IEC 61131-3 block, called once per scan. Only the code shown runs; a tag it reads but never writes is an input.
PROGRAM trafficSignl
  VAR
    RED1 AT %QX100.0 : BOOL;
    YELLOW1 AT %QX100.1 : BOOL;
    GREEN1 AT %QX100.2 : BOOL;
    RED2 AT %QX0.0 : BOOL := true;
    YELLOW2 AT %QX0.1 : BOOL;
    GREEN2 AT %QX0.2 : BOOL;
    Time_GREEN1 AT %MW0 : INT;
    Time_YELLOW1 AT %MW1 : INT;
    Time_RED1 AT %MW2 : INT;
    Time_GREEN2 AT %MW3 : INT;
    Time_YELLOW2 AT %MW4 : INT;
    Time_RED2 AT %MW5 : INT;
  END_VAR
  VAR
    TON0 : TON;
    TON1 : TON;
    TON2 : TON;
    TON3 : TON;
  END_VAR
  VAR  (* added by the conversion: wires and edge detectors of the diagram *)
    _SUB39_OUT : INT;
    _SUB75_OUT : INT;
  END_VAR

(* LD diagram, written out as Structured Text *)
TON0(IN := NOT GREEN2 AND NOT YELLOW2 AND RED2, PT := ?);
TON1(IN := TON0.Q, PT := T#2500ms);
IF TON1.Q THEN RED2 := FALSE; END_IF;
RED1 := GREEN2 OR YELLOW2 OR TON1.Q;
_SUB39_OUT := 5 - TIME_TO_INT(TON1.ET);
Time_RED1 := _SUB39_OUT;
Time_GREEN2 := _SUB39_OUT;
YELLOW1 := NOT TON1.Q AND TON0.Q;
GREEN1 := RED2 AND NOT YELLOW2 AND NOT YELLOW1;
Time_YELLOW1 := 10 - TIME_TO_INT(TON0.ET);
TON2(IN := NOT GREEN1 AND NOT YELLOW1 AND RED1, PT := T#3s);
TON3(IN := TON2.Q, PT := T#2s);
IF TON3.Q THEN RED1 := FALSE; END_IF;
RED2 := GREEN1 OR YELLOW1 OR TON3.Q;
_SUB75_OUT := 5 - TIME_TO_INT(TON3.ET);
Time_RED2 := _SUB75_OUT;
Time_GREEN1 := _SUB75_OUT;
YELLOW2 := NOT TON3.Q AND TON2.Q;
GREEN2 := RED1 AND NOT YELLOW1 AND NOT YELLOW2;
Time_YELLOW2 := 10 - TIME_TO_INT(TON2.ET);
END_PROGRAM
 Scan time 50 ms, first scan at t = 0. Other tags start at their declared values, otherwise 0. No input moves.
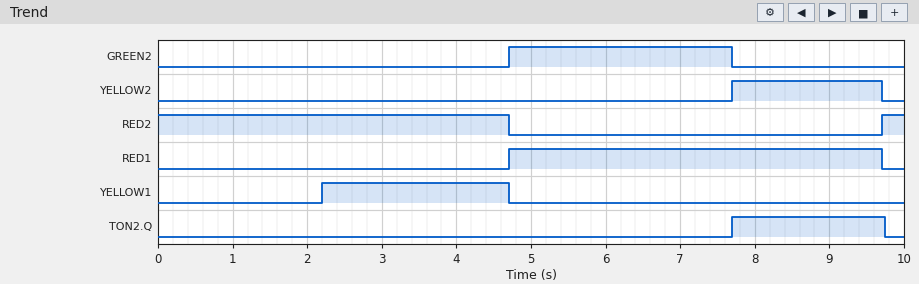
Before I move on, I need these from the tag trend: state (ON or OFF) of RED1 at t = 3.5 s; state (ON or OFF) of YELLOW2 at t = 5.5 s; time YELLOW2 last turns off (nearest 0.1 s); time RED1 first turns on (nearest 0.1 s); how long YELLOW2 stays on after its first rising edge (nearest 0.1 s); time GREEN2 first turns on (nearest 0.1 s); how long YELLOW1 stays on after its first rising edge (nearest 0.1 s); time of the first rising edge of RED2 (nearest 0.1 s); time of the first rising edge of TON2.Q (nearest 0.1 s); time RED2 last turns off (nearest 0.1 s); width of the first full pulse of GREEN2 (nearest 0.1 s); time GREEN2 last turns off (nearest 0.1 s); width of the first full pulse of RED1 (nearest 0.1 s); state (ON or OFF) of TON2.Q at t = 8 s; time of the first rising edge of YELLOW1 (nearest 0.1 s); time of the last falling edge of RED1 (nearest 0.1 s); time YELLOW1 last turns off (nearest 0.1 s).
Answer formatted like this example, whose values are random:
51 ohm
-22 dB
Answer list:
OFF
OFF
9.7 s
4.7 s
2.0 s
4.7 s
2.5 s
9.7 s
7.7 s
4.7 s
3.0 s
7.7 s
5.0 s
ON
2.2 s
9.7 s
4.7 s
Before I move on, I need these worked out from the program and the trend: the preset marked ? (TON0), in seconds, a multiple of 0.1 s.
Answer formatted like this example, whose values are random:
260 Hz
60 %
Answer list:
2.2 s
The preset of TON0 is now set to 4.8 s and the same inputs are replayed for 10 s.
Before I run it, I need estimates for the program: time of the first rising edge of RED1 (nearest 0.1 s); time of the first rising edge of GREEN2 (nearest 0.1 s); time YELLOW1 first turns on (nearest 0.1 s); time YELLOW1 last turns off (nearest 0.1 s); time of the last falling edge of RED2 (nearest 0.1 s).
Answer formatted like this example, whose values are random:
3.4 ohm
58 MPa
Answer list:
7.3 s
7.3 s
4.8 s
7.3 s
7.3 s
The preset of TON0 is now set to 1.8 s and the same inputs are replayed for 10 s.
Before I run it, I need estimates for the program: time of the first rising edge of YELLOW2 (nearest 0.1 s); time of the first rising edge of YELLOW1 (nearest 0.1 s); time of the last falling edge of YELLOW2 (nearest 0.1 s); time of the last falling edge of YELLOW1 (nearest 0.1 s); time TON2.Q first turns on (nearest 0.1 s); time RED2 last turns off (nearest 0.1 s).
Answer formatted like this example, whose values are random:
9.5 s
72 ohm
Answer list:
7.3 s
1.8 s
9.3 s
4.3 s
7.3 s
4.3 s
